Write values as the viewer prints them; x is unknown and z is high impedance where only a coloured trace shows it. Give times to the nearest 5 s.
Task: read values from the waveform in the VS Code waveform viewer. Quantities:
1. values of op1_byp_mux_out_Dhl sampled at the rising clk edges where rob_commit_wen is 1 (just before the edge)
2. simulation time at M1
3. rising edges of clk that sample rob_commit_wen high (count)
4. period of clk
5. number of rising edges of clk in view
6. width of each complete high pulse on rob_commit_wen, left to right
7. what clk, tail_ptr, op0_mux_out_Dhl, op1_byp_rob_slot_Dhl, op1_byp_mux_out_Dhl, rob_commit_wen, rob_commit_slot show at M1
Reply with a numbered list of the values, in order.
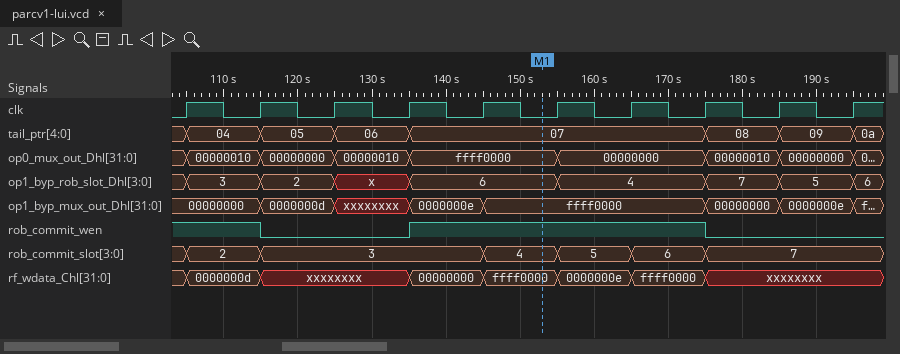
1. 00000000, 00000000, 0000000e, ffff0000, ffff0000, ffff0000
2. 155 s
3. 6
4. 10 s
5. 10
6. 40 s
7. clk=0, tail_ptr=07, op0_mux_out_Dhl=ffff0000, op1_byp_rob_slot_Dhl=6, op1_byp_mux_out_Dhl=ffff0000, rob_commit_wen=1, rob_commit_slot=4
